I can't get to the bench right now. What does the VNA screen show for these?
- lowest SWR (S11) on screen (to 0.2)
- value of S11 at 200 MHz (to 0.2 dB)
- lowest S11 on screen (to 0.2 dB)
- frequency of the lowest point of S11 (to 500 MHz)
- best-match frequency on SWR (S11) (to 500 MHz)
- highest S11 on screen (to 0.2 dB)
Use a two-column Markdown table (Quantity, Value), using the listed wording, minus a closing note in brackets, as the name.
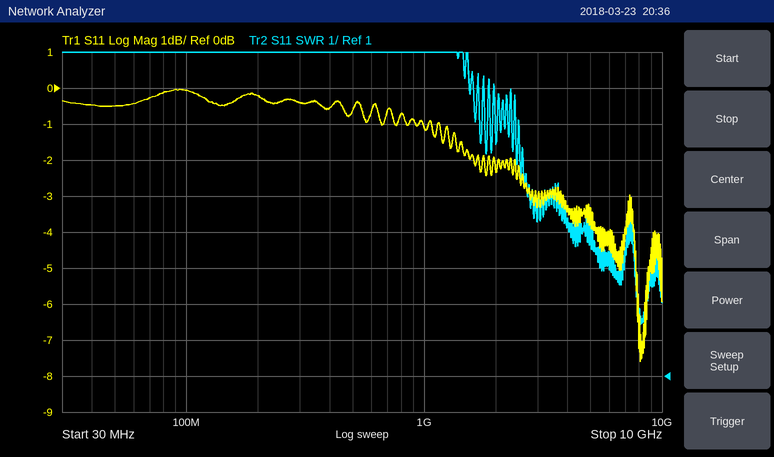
| Quantity | Value |
|---|---|
| lowest SWR (S11) on screen | 2.4 |
| value of S11 at 200 MHz | -0.2 dB |
| lowest S11 on screen | -7.6 dB |
| frequency of the lowest point of S11 | 8.0 GHz |
| best-match frequency on SWR (S11) | 8.0 GHz |
| highest S11 on screen | 0.0 dB |
